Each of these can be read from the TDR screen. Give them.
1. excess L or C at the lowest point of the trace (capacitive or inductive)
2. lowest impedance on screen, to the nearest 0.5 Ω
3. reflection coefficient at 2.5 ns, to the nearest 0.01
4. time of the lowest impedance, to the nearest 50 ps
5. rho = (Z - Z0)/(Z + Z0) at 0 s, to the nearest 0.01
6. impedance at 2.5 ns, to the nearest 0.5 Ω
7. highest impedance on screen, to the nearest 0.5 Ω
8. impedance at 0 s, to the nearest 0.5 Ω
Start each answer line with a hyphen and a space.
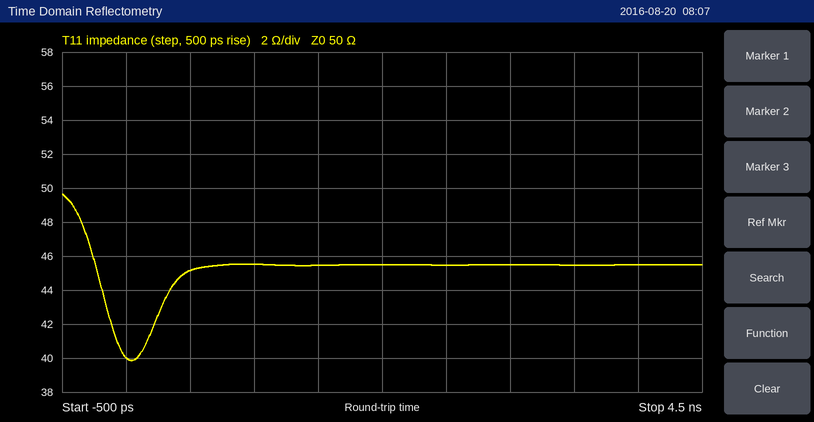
- capacitive
- 40.0 Ω
- -0.05
- 50 ps
- -0.11
- 45.5 Ω
- 49.5 Ω
- 40.0 Ω
